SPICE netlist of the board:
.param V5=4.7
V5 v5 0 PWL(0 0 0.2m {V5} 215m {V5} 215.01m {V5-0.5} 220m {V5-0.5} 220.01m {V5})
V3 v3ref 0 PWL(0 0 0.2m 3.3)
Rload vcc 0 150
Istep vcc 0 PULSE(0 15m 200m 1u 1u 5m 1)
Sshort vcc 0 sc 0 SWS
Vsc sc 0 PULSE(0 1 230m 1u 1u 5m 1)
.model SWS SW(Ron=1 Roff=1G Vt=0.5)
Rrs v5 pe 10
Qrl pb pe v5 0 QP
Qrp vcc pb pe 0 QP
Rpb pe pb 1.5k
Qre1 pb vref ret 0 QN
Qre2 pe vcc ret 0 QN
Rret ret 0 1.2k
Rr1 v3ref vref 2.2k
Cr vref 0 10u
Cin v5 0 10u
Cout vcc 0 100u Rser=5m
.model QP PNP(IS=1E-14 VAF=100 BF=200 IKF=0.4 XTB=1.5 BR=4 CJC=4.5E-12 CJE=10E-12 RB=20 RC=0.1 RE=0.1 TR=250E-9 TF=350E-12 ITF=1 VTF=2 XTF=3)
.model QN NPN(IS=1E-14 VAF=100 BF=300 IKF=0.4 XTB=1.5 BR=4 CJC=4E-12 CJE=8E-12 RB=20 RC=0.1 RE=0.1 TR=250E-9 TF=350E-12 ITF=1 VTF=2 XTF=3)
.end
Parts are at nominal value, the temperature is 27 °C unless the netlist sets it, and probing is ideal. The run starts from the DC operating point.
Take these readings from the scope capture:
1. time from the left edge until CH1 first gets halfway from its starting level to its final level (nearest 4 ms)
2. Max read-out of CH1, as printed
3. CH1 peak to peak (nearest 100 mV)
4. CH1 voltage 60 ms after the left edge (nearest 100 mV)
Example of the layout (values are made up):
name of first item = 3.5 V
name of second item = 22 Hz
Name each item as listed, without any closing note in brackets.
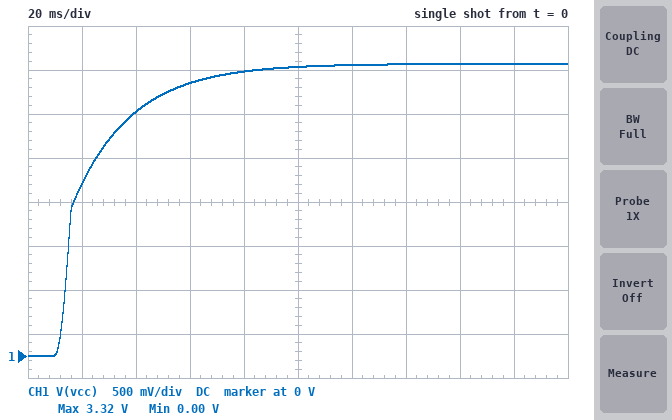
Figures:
time from the left edge until CH1 first gets halfway from its starting level to its final level = 16 ms
Max read-out of CH1, as printed = 3.32 V
CH1 peak to peak = 3.3 V
CH1 voltage 60 ms after the left edge = 3.1 V
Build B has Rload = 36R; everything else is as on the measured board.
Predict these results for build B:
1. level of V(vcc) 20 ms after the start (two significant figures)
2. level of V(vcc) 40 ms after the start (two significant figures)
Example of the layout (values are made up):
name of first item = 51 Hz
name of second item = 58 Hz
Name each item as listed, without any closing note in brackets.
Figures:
level of V(vcc) 20 ms after the start = 1.8 V
level of V(vcc) 40 ms after the start = 2.3 V
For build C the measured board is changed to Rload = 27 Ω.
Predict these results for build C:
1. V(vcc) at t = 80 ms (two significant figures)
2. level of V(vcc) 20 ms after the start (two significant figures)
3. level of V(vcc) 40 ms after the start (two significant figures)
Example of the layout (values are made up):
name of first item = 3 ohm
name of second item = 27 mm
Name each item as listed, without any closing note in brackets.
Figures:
V(vcc) at t = 80 ms = 1.8 V
level of V(vcc) 20 ms after the start = 1.5 V
level of V(vcc) 40 ms after the start = 1.7 V
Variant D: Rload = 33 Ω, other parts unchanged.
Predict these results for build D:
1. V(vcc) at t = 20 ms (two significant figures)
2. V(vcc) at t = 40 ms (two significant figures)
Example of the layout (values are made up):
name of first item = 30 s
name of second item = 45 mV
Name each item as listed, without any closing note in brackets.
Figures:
V(vcc) at t = 20 ms = 1.7 V
V(vcc) at t = 40 ms = 2.1 V
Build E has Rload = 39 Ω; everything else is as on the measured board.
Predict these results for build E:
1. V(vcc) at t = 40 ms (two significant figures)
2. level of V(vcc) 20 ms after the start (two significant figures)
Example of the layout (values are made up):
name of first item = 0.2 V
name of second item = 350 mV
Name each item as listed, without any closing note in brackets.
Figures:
V(vcc) at t = 40 ms = 2.5 V
level of V(vcc) 20 ms after the start = 1.9 V
